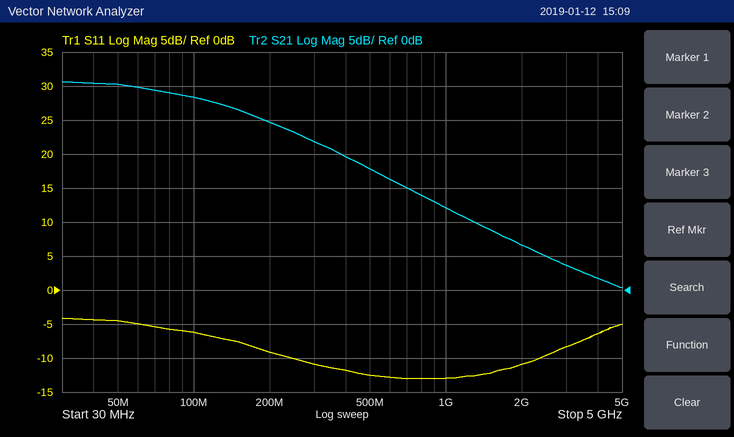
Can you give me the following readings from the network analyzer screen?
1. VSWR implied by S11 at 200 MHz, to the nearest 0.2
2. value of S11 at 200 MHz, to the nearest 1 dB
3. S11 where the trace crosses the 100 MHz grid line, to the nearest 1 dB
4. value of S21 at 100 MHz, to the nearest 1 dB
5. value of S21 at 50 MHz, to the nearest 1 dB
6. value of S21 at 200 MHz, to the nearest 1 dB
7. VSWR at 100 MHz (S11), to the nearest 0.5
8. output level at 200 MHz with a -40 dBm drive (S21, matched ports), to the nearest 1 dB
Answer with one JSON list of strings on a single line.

["2.0", "-9 dB", "-6 dB", "28 dB", "30 dB", "25 dB", "3.0", "-15 dBm"]
